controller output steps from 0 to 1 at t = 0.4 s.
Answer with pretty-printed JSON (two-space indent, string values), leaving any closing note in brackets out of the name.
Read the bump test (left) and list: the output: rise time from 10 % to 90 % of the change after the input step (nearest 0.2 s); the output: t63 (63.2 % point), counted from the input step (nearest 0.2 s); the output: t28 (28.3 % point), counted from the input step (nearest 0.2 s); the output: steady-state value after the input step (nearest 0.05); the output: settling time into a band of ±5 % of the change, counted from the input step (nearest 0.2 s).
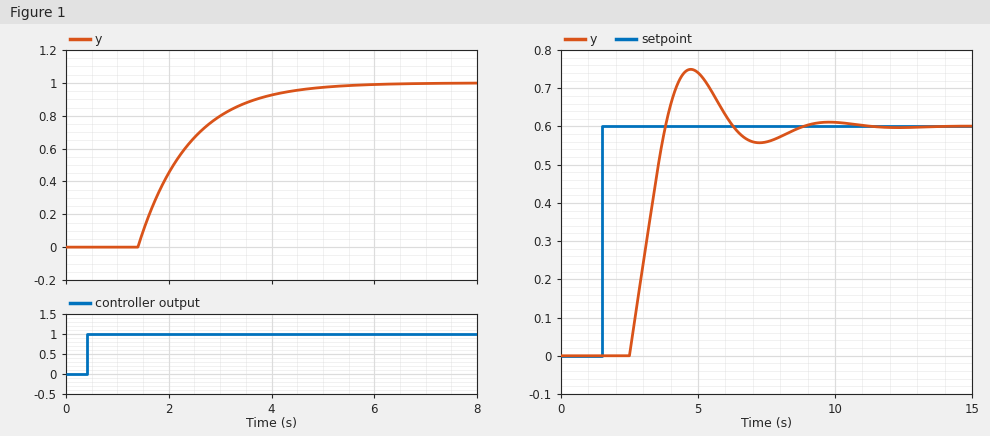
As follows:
{
  "the output: rise time from 10 % to 90 % of the change after the input step": "2.2 s",
  "the output: t63 (63.2 % point), counted from the input step": "2.0 s",
  "the output: t28 (28.3 % point), counted from the input step": "1.4 s",
  "the output: steady-state value after the input step": "1.00",
  "the output: settling time into a band of ±5 % of the change, counted from the input step": "4.0 s"
}
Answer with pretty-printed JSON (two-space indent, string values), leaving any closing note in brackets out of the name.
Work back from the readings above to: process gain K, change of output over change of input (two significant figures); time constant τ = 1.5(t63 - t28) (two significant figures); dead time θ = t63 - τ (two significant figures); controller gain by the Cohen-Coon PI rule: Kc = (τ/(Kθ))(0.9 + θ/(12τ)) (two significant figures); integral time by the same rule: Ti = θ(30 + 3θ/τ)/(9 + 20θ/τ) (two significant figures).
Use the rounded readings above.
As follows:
{
  "process gain K, change of output over change of input": "1.0",
  "time constant τ = 1.5(t63 - t28)": "0.90 s",
  "dead time θ = t63 - τ": "1.1 s",
  "controller gain by the Cohen-Coon PI rule: Kc = (τ/(Kθ))(0.9 + θ/(12τ))": "0.82",
  "integral time by the same rule: Ti = θ(30 + 3θ/τ)/(9 + 20θ/τ)": "1.1 s"
}
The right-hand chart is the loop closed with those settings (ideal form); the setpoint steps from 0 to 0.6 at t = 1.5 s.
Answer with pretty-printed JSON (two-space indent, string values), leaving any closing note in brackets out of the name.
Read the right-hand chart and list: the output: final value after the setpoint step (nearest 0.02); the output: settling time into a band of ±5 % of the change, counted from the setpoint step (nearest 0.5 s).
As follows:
{
  "the output: final value after the setpoint step": "0.60",
  "the output: settling time into a band of ±5 % of the change, counted from the setpoint step": "6.5 s"
}
